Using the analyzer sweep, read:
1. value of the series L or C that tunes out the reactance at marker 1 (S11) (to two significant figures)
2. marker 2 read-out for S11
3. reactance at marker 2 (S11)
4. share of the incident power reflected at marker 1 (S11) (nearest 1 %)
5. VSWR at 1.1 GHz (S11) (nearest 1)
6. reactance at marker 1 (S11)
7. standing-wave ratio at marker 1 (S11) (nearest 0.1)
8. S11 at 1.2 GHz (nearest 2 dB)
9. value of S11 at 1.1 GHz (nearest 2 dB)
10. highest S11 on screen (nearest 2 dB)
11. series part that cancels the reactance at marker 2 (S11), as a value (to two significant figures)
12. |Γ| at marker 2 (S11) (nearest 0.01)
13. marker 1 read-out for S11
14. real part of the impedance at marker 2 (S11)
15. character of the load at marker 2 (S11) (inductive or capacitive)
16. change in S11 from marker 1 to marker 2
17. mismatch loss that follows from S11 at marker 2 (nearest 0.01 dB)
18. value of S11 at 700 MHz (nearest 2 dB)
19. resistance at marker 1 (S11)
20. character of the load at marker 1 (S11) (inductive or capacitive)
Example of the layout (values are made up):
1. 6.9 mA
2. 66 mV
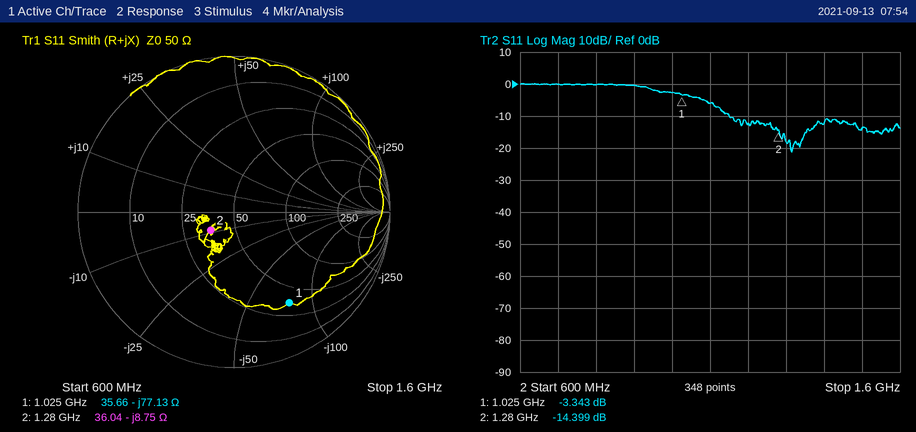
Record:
1. 12 nH
2. -14.399 dB
3. -8.75 Ω
4. 46 %
5. 3
6. -77.13 Ω
7. 5.3
8. -12 dB
9. -6 dB
10. 0 dB
11. 1.1 nH
12. 0.19
13. -3.343 dB
14. 36.04 Ω
15. capacitive
16. -11.056 dB
17. 0.16 dB
18. 0 dB
19. 35.66 Ω
20. capacitive
